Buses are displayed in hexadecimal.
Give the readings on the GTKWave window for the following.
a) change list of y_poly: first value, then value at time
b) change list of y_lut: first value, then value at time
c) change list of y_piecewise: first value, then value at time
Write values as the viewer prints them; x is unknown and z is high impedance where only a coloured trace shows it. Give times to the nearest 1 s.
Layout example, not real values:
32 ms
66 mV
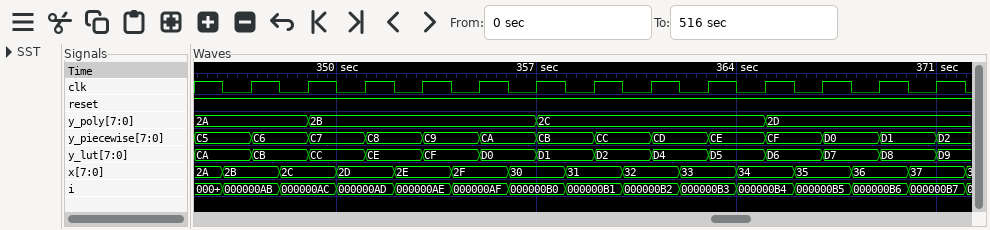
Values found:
2A, 2B at 349 s, 2C at 357 s, 2D at 365 s
CA, CB at 347 s, CC at 349 s, CE at 351 s, CF at 353 s, D0 at 355 s, D1 at 357 s, D2 at 359 s, D4 at 361 s, D5 at 363 s, D6 at 365 s, D7 at 367 s, D8 at 369 s, D9 at 371 s
C5, C6 at 347 s, C7 at 349 s, C8 at 351 s, C9 at 353 s, CA at 355 s, CB at 357 s, CC at 359 s, CD at 361 s, CE at 363 s, CF at 365 s, D0 at 367 s, D1 at 369 s, D2 at 371 s
